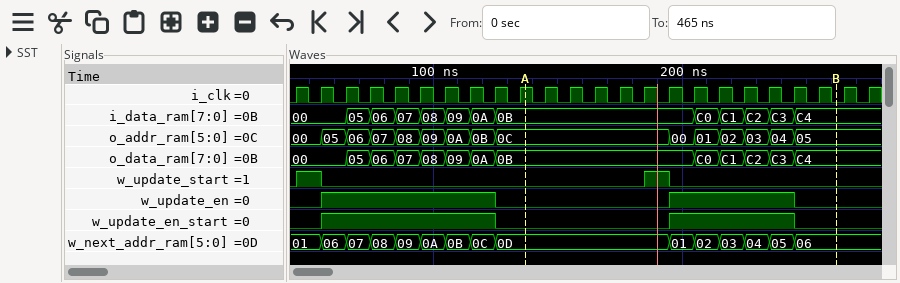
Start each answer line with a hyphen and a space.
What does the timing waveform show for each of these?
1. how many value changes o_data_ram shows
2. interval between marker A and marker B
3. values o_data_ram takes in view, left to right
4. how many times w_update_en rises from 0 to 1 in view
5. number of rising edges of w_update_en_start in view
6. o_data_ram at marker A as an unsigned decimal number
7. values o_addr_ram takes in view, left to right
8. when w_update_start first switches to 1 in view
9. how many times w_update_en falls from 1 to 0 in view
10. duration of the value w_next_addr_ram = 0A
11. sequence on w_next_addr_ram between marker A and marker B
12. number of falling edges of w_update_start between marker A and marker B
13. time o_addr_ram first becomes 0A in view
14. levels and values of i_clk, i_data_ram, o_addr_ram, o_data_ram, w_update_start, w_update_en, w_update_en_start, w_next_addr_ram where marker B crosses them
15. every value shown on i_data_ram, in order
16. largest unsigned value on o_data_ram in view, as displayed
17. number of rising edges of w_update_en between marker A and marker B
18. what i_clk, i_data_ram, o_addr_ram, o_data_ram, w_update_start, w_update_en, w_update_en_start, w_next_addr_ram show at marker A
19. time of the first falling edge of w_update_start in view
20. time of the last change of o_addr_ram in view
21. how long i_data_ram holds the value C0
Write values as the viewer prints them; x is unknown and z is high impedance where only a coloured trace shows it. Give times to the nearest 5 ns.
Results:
- 12
- 125 ns
- 00, 05, 06, 07, 08, 09, 0A, 0B, C0, C1, C2, C3, C4
- 2
- 2
- 11
- 00, 05, 06, 07, 08, 09, 0A, 0B, 0C, 00, 01, 02, 03, 04, 05
- 45 ns
- 2
- 10 ns
- 0D, 01, 02, 03, 04, 05, 06
- 1
- 105 ns
- i_clk=0, i_data_ram=C4, o_addr_ram=05, o_data_ram=C4, w_update_start=0, w_update_en=0, w_update_en_start=0, w_next_addr_ram=06
- 00, 05, 06, 07, 08, 09, 0A, 0B, C0, C1, C2, C3, C4
- C4
- 1
- i_clk=1, i_data_ram=0B, o_addr_ram=0C, o_data_ram=0B, w_update_start=0, w_update_en=0, w_update_en_start=0, w_next_addr_ram=0D
- 55 ns
- 245 ns
- 10 ns
